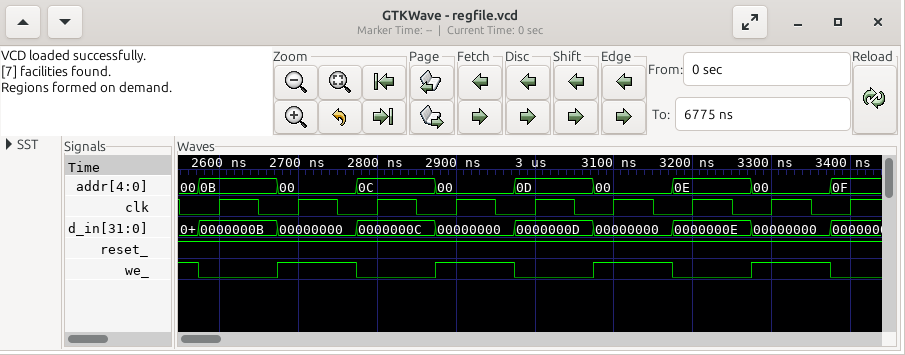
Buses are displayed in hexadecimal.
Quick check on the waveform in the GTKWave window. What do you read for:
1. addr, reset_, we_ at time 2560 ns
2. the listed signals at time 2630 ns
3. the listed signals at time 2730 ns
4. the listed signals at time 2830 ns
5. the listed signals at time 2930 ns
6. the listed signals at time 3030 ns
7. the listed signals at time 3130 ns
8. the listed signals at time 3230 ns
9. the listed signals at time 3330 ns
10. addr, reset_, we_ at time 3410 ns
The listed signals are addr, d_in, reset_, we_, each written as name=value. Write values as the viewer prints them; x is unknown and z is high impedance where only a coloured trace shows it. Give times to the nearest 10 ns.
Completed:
addr=00, reset_=1, we_=1
addr=0B, d_in=0000000B, reset_=1, we_=0
addr=00, d_in=00000000, reset_=1, we_=1
addr=0C, d_in=0000000C, reset_=1, we_=0
addr=00, d_in=00000000, reset_=1, we_=1
addr=0D, d_in=0000000D, reset_=1, we_=0
addr=00, d_in=00000000, reset_=1, we_=1
addr=0E, d_in=0000000E, reset_=1, we_=0
addr=00, d_in=00000000, reset_=1, we_=1
addr=0F, reset_=1, we_=0
